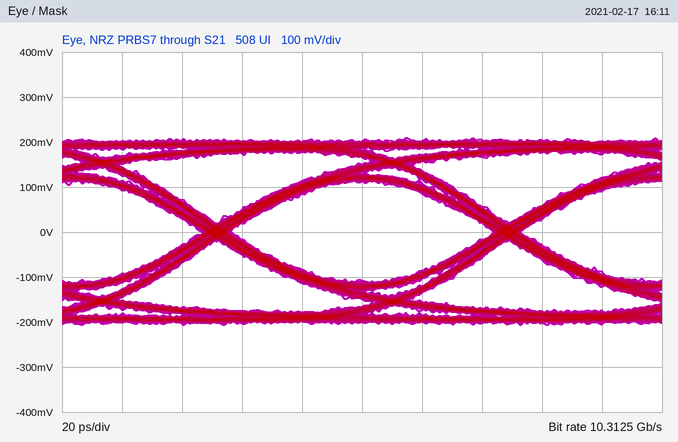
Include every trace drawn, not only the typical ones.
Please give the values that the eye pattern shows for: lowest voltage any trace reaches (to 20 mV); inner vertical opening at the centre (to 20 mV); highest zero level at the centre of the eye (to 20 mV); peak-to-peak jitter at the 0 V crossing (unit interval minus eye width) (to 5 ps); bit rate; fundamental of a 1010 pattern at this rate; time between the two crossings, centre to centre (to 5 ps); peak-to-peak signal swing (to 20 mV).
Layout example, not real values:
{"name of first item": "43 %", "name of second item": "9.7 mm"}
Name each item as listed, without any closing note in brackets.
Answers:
{"lowest voltage any trace reaches": "-200 mV", "inner vertical opening at the centre": "220 mV", "highest zero level at the centre of the eye": "-100 mV", "peak-to-peak jitter at the 0 V crossing (unit interval minus eye width)": "10 ps", "bit rate": "10.3125 Gb/s", "fundamental of a 1010 pattern at this rate": "5.15625 GHz", "time between the two crossings, centre to centre": "95 ps", "peak-to-peak signal swing": "420 mV"}
